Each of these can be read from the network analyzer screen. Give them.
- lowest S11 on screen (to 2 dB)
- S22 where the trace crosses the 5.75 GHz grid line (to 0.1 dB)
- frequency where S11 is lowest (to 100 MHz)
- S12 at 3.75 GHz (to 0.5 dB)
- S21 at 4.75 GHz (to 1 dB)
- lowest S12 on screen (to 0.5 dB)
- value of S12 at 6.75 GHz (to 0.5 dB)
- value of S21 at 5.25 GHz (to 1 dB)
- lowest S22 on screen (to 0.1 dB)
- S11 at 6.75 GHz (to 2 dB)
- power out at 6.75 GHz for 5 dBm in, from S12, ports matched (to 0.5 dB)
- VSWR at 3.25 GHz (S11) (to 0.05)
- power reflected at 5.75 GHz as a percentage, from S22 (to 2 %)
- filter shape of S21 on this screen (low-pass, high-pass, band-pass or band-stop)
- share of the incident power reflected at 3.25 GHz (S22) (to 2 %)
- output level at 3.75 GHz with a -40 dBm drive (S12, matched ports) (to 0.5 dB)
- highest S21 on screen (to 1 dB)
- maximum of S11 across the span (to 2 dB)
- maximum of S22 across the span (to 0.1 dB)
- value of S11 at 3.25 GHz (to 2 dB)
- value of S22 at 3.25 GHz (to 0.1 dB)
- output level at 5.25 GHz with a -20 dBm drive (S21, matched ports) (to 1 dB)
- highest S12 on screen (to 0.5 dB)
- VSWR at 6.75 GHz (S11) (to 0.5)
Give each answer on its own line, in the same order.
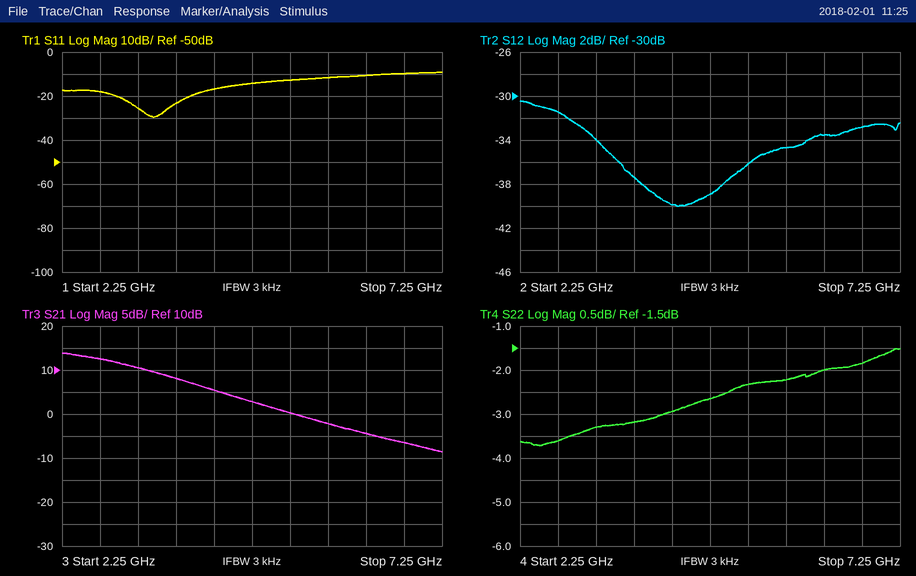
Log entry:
-30 dB
-2.2 dB
3.5 GHz
-37.5 dB
3 dB
-40.0 dB
-33.0 dB
0 dB
-3.7 dB
-10 dB
-28.0 dBm
1.10
60 %
low-pass
46 %
-77.5 dBm
14 dB
-10 dB
-1.5 dB
-26 dB
-3.3 dB
-20 dBm
-30.5 dB
2.0
